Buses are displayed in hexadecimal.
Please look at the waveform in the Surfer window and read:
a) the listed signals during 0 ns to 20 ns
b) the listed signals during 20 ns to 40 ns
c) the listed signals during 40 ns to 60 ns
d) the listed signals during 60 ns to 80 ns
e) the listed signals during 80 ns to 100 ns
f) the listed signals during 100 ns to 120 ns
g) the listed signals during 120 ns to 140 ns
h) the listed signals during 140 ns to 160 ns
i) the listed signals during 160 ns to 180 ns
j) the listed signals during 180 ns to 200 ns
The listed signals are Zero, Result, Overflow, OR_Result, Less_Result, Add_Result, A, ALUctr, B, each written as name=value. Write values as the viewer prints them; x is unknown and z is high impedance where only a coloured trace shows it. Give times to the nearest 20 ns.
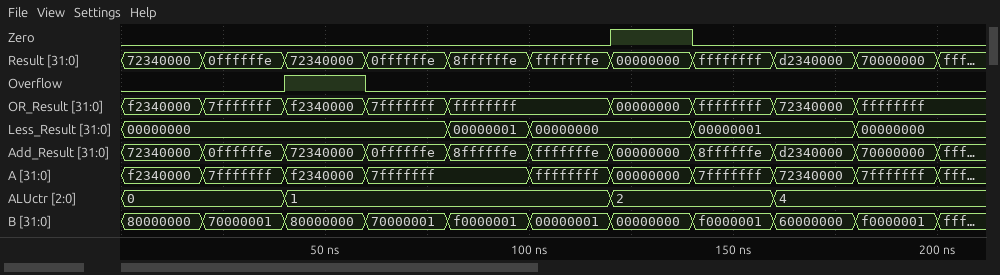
Zero=0, Result=72340000, Overflow=0, OR_Result=f2340000, Less_Result=00000000, Add_Result=72340000, A=f2340000, ALUctr=0, B=80000000
Zero=0, Result=0ffffffe, Overflow=0, OR_Result=7fffffff, Less_Result=00000000, Add_Result=0ffffffe, A=7fffffff, ALUctr=0, B=70000001
Zero=0, Result=72340000, Overflow=1, OR_Result=f2340000, Less_Result=00000000, Add_Result=72340000, A=f2340000, ALUctr=1, B=80000000
Zero=0, Result=0ffffffe, Overflow=0, OR_Result=7fffffff, Less_Result=00000000, Add_Result=0ffffffe, A=7fffffff, ALUctr=1, B=70000001
Zero=0, Result=8ffffffe, Overflow=0, OR_Result=ffffffff, Less_Result=00000001, Add_Result=8ffffffe, A=7fffffff, ALUctr=1, B=f0000001
Zero=0, Result=fffffffe, Overflow=0, OR_Result=ffffffff, Less_Result=00000000, Add_Result=fffffffe, A=ffffffff, ALUctr=1, B=00000001
Zero=1, Result=00000000, Overflow=0, OR_Result=00000000, Less_Result=00000000, Add_Result=00000000, A=00000000, ALUctr=2, B=00000000
Zero=0, Result=ffffffff, Overflow=0, OR_Result=ffffffff, Less_Result=00000001, Add_Result=8ffffffe, A=7fffffff, ALUctr=2, B=f0000001
Zero=0, Result=d2340000, Overflow=0, OR_Result=72340000, Less_Result=00000001, Add_Result=d2340000, A=72340000, ALUctr=4, B=60000000
Zero=0, Result=70000000, Overflow=0, OR_Result=ffffffff, Less_Result=00000000, Add_Result=70000000, A=7fffffff, ALUctr=4, B=f0000001
